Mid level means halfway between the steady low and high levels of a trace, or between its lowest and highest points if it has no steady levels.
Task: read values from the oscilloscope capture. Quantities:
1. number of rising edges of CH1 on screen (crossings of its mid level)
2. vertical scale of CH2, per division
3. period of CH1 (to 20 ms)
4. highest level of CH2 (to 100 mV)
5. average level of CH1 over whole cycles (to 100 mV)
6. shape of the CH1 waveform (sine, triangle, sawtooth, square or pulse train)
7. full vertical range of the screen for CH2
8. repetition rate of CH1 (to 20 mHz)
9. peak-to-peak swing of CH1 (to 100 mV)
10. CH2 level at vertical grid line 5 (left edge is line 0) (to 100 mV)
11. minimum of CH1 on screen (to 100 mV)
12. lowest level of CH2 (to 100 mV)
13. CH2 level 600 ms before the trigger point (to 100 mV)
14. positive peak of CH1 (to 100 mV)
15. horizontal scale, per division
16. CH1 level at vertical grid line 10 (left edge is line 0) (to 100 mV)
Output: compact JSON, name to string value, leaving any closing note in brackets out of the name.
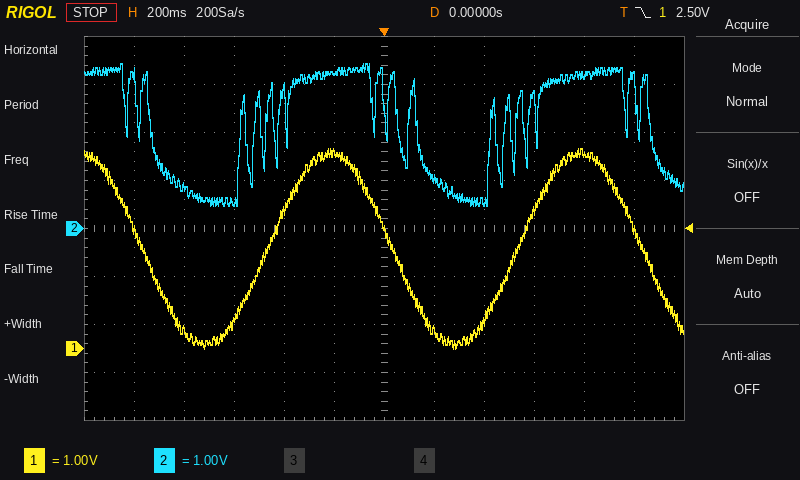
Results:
{"number of rising edges of CH1 on screen": "2", "vertical scale of CH2, per division": "1 V", "period of CH1": "1.00 s", "highest level of CH2": "3.4 V", "average level of CH1 over whole cycles": "2.1 V", "shape of the CH1 waveform": "sine", "full vertical range of the screen for CH2": "8 V", "repetition rate of CH1": "1.00 Hz", "peak-to-peak swing of CH1": "4.2 V", "CH2 level at vertical grid line 5 (left edge is line 0)": "3.2 V", "minimum of CH1 on screen": "0.0 V", "lowest level of CH2": "500 mV", "CH2 level 600 ms before the trigger point": "600 mV", "positive peak of CH1": "4.2 V", "horizontal scale, per division": "200 ms", "CH1 level at vertical grid line 10 (left edge is line 0)": "4.1 V"}
